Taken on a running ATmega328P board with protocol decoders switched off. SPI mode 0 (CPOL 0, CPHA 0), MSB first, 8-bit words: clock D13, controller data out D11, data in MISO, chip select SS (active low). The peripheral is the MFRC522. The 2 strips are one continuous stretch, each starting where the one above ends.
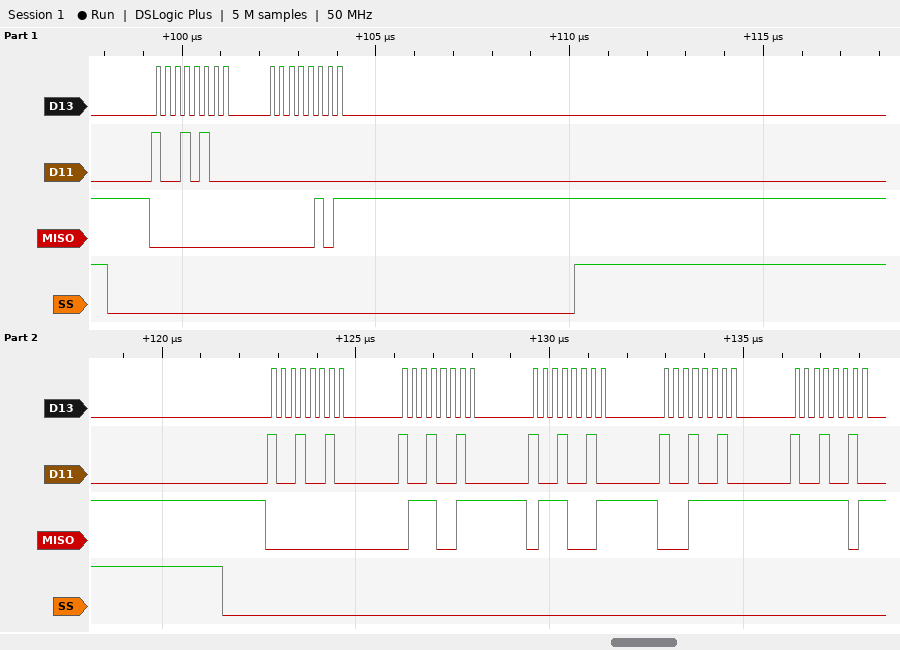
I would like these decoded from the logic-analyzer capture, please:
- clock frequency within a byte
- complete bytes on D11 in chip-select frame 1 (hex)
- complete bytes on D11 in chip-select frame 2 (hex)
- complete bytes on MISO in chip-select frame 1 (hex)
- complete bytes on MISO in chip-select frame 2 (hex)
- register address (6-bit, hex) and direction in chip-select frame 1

4 MHz
94 00
92 92 92 92 92
00 05
00 73 71 1F FD
0x0A read
